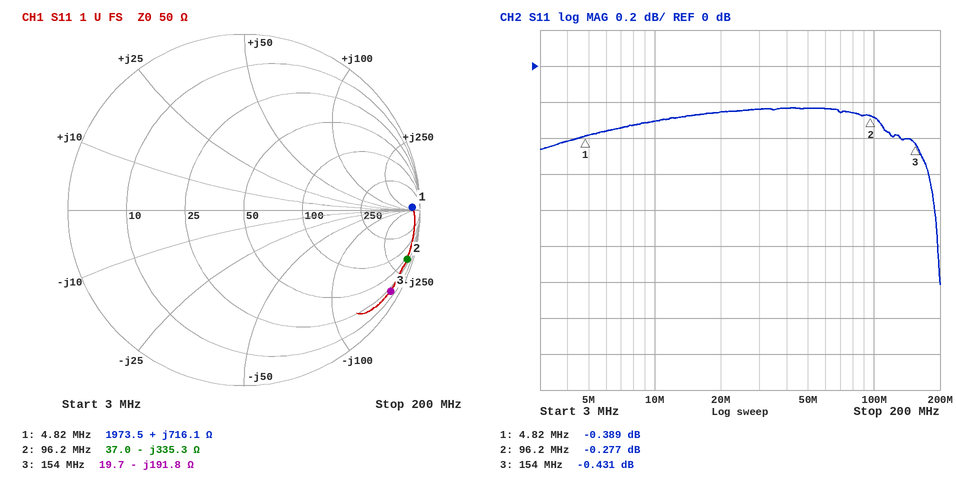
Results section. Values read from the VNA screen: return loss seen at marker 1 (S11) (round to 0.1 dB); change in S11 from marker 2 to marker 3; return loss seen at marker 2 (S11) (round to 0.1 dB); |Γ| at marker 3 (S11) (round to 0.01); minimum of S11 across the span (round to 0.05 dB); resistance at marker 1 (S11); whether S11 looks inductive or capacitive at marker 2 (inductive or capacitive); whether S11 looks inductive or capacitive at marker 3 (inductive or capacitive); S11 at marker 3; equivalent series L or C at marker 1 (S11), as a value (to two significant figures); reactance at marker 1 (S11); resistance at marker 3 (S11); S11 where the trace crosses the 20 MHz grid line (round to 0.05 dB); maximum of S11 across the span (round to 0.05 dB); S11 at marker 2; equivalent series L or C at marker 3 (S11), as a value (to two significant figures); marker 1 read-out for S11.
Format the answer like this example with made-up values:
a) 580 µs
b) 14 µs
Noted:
a) 0.4 dB
b) -0.154 dB
c) 0.3 dB
d) 0.95
e) -1.20 dB
f) 1973.5 Ω
g) capacitive
h) capacitive
i) -0.431 dB
j) 24 µH
k) +716.1 Ω
l) 19.7 Ω
m) -0.25 dB
n) -0.25 dB
o) -0.277 dB
p) 5.4 pF
q) -0.389 dB
